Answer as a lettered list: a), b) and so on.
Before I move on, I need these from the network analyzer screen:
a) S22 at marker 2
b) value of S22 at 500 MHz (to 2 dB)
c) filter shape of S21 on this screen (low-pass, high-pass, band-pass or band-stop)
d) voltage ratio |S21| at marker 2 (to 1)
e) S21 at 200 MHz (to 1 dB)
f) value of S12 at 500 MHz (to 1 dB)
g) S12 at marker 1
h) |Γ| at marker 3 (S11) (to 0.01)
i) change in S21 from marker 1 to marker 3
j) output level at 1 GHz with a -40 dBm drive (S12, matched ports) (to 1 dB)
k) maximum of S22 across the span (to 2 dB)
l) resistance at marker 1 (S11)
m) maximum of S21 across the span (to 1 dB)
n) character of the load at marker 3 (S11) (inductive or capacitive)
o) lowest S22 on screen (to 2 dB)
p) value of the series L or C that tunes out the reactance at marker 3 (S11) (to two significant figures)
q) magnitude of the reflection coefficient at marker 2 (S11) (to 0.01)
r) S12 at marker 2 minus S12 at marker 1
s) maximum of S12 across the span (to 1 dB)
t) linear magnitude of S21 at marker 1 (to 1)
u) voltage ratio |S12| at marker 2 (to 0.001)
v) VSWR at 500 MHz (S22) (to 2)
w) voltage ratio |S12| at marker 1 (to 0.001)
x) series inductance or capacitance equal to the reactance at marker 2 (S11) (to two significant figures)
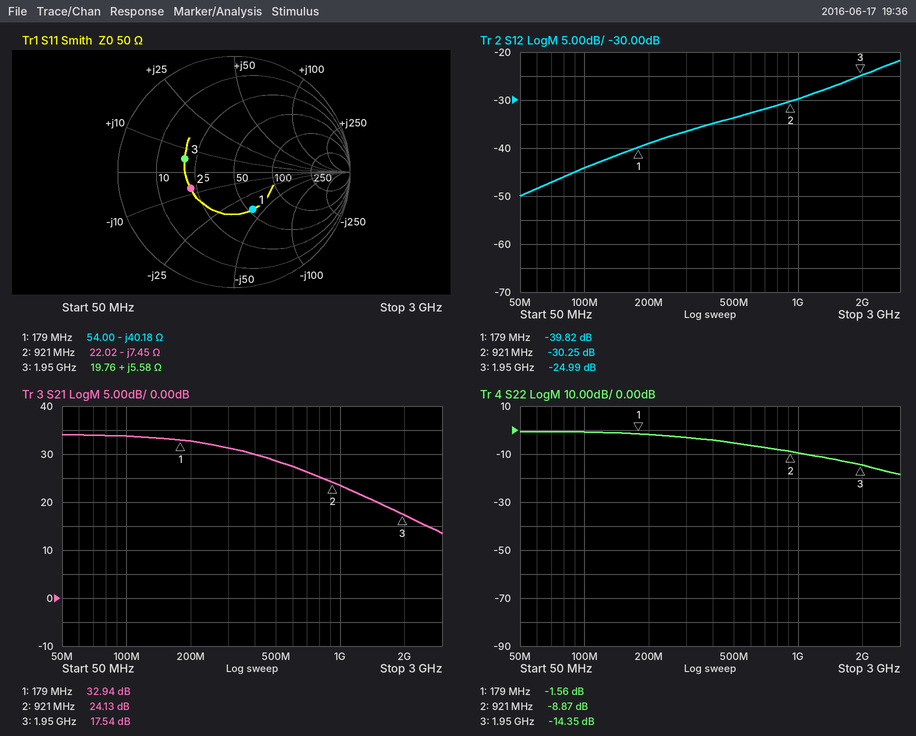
a) -8.87 dB
b) -6 dB
c) low-pass
d) 16
e) 33 dB
f) -34 dB
g) -39.82 dB
h) 0.44
i) -15.40 dB
j) -70 dBm
k) 0 dB
l) 54.00 Ω
m) 34 dB
n) inductive
o) -18 dB
p) 15 pF
q) 0.40
r) 9.57 dB
s) -22 dB
t) 44
u) 0.031
v) 4
w) 0.010
x) 23 pF
